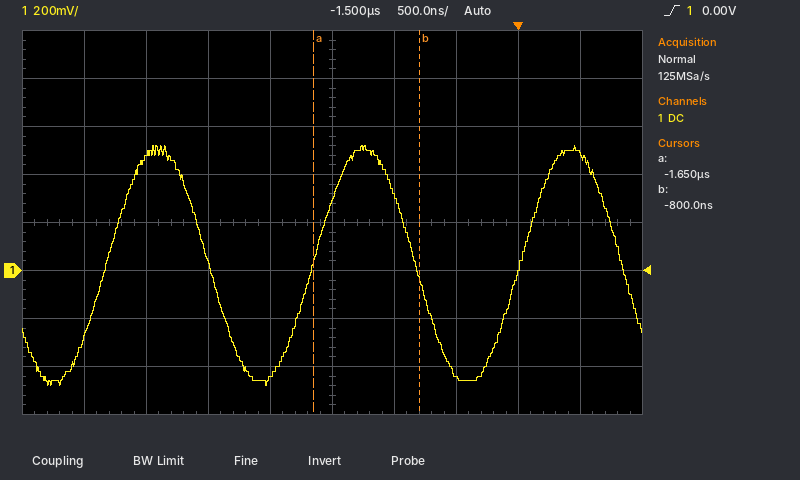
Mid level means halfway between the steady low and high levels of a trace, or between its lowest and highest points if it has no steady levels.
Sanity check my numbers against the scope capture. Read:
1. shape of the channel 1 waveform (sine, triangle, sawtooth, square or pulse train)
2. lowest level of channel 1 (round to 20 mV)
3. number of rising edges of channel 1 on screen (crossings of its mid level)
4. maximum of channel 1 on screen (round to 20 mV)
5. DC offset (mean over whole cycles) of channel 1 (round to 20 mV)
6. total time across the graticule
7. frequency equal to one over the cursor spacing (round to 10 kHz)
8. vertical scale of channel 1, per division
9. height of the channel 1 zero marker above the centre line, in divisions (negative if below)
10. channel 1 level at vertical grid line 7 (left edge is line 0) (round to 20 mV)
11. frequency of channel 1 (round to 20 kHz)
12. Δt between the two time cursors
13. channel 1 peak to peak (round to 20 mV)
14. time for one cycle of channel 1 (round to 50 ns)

sine
-480 mV
3
520 mV
20 mV
5 µs
1.18 MHz
200 mV
-1.0 div
-440 mV
600 kHz
850 ns
1.00 V
1.65 µs
